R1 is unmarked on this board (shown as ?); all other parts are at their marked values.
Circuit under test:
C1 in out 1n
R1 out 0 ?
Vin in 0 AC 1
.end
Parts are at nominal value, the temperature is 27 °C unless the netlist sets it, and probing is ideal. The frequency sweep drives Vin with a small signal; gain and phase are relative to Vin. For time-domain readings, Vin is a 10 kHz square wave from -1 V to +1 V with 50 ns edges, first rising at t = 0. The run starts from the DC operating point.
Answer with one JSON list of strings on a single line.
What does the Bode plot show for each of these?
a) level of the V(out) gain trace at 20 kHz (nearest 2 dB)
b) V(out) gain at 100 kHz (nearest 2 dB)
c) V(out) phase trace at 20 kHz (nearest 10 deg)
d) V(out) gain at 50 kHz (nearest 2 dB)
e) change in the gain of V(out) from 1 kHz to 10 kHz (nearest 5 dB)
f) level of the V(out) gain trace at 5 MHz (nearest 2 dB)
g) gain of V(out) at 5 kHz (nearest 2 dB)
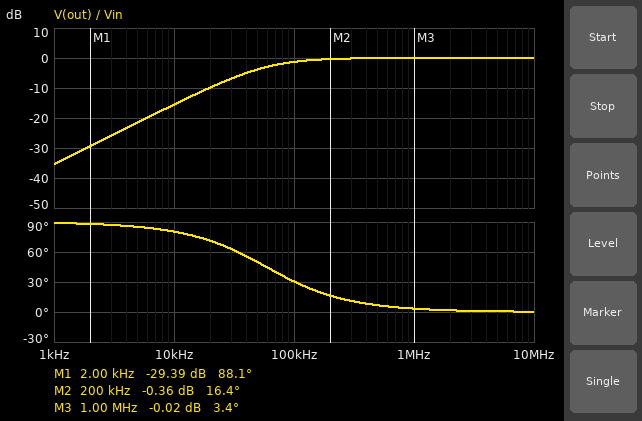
["-10 dB", "-2 dB", "70 deg", "-4 dB", "20 dB", "0 dB", "-22 dB"]
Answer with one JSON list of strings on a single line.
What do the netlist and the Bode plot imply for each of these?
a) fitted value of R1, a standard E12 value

["2.7 kΩ"]
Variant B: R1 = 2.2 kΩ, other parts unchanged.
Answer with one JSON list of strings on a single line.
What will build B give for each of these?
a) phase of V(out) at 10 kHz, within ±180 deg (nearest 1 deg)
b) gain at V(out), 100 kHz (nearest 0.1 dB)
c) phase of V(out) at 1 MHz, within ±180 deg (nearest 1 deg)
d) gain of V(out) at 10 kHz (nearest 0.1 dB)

["82 deg", "-1.8 dB", "4 deg", "-17.3 dB"]
